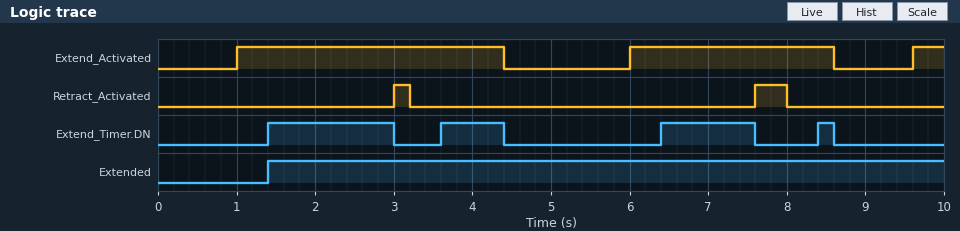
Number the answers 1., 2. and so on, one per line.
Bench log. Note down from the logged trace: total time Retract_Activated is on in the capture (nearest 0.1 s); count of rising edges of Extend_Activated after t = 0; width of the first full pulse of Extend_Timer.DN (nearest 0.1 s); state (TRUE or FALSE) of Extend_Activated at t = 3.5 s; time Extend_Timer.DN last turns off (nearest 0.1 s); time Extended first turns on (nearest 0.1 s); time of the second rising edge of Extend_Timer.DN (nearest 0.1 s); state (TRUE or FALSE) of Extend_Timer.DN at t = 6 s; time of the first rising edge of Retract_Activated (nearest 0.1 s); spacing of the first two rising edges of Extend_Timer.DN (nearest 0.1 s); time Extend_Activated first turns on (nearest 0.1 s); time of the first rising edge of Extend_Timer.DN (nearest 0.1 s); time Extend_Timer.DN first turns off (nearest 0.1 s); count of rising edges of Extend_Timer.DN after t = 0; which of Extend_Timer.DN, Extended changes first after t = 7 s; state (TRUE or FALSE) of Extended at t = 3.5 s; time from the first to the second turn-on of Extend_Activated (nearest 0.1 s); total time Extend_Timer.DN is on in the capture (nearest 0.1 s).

1. 0.6 s
2. 3
3. 1.6 s
4. TRUE
5. 8.6 s
6. 1.4 s
7. 3.6 s
8. FALSE
9. 3.0 s
10. 2.2 s
11. 1.0 s
12. 1.4 s
13. 3.0 s
14. 4
15. Extend_Timer.DN
16. TRUE
17. 5.0 s
18. 3.8 s
